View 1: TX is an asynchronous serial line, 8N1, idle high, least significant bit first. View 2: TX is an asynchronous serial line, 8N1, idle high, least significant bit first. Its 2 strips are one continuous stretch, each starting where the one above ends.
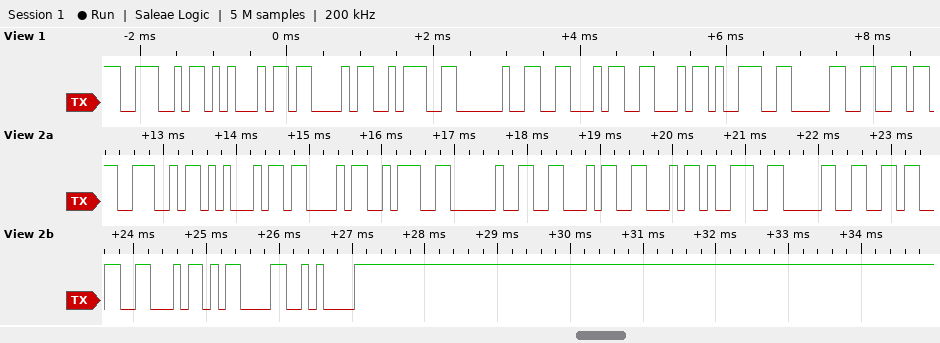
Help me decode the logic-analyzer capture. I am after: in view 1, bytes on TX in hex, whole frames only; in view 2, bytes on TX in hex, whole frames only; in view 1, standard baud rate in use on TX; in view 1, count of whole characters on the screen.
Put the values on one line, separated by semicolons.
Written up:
4E 45 43 3A 20 46 46 39 30; 4E 45 43 3A 20 46 46 39 30 36 46 0D 0A; 9600 baud; 9
